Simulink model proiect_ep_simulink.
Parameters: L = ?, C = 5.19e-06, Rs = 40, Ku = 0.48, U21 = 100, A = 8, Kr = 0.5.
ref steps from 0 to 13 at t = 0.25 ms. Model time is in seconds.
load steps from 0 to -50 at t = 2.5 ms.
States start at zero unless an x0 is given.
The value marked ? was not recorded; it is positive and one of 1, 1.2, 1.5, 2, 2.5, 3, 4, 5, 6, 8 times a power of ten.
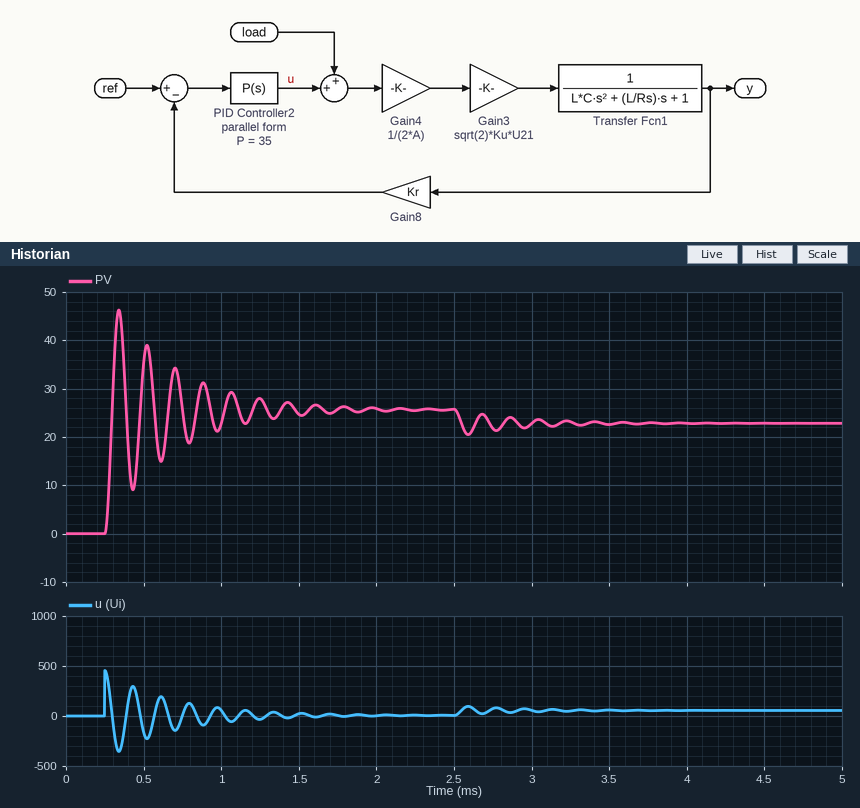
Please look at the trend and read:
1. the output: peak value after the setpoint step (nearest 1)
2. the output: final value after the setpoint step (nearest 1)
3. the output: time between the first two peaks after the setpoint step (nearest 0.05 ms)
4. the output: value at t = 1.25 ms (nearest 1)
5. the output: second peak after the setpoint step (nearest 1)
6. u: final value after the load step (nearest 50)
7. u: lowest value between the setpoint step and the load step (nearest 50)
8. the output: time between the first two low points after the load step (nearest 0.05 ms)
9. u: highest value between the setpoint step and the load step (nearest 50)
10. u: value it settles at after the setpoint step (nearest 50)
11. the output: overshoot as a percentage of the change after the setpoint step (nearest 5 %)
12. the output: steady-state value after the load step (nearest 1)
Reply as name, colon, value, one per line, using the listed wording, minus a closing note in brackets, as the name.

the output: peak value after the setpoint step: 46
the output: final value after the setpoint step: 26
the output: time between the first two peaks after the setpoint step: 0.20 ms
the output: value at t = 1.25 ms: 28
the output: second peak after the setpoint step: 39
u: final value after the load step: 50
u: lowest value between the setpoint step and the load step: -350
the output: time between the first two low points after the load step: 0.20 ms
u: highest value between the setpoint step and the load step: 450
u: value it settles at after the setpoint step: 0
the output: overshoot as a percentage of the change after the setpoint step: 80 %
the output: steady-state value after the load step: 23
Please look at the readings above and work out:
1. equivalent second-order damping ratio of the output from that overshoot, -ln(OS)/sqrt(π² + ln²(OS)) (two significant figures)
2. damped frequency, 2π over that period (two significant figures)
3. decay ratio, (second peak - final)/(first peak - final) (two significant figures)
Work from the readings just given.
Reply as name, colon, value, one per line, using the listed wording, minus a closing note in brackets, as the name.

equivalent second-order damping ratio of the output from that overshoot, -ln(OS)/sqrt(π² + ln²(OS)): 0.071
damped frequency, 2π over that period: 31 rad/ms
decay ratio, (second peak - final)/(first peak - final): 0.65
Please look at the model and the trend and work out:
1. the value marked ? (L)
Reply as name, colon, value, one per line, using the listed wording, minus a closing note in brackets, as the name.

the value marked ?: 0.012
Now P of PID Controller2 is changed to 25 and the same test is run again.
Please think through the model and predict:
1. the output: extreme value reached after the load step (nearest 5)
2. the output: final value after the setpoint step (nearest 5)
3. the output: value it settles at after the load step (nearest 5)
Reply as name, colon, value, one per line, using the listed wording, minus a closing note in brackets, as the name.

the output: extreme value reached after the load step: 20
the output: final value after the setpoint step: 25
the output: value it settles at after the load step: 20
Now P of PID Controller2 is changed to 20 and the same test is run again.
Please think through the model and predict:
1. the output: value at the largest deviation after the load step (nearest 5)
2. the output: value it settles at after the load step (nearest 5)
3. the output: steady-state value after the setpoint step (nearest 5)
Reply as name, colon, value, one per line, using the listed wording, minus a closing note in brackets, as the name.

the output: value at the largest deviation after the load step: 15
the output: value it settles at after the load step: 20
the output: steady-state value after the setpoint step: 25
